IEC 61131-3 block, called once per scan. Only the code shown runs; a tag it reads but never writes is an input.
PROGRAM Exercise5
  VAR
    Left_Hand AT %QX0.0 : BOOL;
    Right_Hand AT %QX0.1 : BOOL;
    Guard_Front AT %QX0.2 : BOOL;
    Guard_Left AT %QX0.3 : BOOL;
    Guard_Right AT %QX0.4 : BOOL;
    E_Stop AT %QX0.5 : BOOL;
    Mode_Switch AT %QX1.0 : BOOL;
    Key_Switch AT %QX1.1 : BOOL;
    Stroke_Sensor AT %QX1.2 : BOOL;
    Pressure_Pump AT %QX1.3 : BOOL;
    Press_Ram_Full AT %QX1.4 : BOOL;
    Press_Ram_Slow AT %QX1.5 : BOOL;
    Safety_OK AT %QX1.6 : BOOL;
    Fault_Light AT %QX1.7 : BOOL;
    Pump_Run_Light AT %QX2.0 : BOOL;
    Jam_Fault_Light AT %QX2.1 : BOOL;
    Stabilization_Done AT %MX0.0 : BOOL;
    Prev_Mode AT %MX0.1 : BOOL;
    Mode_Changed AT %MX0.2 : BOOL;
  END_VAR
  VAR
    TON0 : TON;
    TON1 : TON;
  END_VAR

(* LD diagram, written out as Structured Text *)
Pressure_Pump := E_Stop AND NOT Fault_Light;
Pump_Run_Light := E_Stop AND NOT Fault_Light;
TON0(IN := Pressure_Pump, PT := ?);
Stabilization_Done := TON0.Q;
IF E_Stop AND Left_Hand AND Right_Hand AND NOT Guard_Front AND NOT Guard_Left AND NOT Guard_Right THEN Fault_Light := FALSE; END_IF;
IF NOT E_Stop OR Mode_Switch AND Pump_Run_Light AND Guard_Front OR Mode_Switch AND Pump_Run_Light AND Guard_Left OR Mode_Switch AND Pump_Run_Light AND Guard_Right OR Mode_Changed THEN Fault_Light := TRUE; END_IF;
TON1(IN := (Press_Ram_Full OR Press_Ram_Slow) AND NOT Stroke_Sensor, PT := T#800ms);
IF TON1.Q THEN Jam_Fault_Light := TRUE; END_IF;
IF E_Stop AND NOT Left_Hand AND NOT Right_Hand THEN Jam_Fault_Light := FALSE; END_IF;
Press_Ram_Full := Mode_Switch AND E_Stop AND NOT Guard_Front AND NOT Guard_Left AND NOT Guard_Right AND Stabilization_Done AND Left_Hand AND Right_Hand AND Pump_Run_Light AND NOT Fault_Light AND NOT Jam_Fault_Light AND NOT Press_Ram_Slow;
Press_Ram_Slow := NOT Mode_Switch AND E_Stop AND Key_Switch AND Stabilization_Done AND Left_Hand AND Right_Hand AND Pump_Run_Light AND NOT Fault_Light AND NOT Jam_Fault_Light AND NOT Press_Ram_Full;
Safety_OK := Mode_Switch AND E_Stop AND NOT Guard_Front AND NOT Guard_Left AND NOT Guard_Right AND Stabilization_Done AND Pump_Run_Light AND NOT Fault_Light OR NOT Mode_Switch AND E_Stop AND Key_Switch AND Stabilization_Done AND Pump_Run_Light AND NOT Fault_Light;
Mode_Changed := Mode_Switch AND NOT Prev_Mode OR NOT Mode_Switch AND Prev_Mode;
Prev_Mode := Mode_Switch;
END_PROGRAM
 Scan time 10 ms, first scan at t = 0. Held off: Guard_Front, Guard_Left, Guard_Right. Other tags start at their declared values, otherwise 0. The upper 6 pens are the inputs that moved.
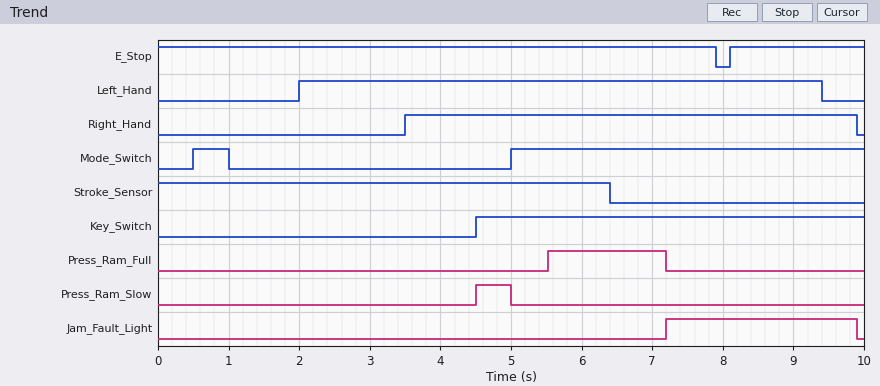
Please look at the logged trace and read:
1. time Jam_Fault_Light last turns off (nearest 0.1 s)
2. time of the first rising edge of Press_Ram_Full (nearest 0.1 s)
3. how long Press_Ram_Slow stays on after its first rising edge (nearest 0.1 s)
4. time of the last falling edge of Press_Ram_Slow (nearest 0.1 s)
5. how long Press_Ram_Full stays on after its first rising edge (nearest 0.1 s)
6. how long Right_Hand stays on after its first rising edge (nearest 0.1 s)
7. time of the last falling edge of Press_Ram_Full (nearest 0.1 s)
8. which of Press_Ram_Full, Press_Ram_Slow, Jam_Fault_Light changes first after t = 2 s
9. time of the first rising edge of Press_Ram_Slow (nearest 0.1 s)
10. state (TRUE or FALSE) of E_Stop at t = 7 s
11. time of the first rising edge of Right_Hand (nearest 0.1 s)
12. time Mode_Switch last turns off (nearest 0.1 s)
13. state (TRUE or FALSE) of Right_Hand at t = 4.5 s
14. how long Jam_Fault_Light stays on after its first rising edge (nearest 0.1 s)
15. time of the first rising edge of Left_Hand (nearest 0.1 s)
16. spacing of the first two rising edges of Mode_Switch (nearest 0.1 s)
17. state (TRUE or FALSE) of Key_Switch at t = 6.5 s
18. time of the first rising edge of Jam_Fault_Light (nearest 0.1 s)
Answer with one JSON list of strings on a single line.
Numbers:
["9.9 s", "5.5 s", "0.5 s", "5.0 s", "1.7 s", "6.4 s", "7.2 s", "Press_Ram_Slow", "4.5 s", "TRUE", "3.5 s", "1.0 s", "TRUE", "2.7 s", "2.0 s", "4.5 s", "TRUE", "7.2 s"]
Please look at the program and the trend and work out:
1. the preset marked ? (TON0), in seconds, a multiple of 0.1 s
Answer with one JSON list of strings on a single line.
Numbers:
["0.5 s"]
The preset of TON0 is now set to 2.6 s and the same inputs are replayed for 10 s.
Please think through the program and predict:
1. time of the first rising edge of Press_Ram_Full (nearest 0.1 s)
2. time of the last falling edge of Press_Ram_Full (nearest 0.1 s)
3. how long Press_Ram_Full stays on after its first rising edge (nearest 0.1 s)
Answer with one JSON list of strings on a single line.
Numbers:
["7.6 s", "7.9 s", "0.3 s"]
